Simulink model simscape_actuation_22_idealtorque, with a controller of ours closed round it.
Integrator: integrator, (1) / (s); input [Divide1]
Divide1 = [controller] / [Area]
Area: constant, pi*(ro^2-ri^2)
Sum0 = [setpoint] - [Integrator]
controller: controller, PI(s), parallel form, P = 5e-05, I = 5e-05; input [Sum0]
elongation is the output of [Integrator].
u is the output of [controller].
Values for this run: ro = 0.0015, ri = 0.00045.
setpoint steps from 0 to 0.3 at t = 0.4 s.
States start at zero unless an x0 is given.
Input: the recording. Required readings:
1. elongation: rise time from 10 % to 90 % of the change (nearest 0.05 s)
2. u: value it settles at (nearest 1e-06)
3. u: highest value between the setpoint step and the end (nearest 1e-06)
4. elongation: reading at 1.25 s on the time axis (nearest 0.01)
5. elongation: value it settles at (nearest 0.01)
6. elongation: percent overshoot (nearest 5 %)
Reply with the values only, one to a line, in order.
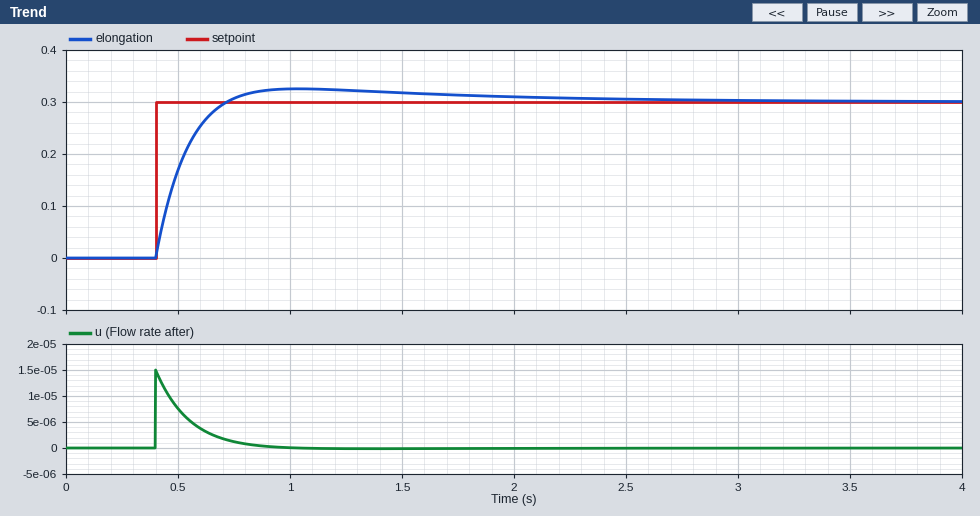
0.20 s
0.000000
0.000015
0.32
0.30
10 %
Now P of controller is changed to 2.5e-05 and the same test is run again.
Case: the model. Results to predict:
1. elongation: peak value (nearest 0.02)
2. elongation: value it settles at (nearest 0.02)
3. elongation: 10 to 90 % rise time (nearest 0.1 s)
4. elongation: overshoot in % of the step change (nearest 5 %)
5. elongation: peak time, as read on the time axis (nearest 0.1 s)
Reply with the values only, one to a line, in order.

0.36
0.30
0.3 s
20 %
1.2 s
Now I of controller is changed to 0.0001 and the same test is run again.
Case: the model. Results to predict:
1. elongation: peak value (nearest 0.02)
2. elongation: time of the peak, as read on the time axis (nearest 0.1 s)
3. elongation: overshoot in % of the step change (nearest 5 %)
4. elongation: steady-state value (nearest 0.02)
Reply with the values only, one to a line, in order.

0.34
0.9 s
15 %
0.30
